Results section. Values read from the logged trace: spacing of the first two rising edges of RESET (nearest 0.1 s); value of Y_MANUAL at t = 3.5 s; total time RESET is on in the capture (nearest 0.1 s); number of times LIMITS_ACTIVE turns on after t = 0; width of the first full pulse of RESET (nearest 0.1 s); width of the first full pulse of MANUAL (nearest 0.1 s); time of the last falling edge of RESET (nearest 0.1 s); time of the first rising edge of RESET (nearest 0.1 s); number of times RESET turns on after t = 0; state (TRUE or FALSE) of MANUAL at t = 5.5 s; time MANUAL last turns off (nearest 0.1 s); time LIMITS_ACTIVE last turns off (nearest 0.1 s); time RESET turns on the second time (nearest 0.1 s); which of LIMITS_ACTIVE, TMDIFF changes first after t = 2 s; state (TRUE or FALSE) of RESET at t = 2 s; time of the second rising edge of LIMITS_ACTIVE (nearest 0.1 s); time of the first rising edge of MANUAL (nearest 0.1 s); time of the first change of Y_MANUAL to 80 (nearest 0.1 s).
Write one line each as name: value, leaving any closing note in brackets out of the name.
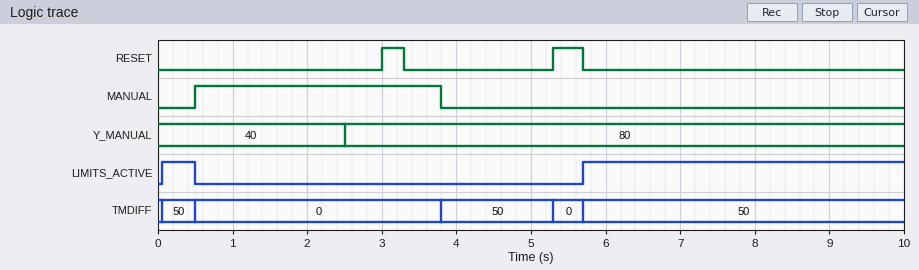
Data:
spacing of the first two rising edges of RESET: 2.3 s
value of Y_MANUAL at t = 3.5 s: 80
total time RESET is on in the capture: 0.7 s
number of times LIMITS_ACTIVE turns on after t = 0: 2
width of the first full pulse of RESET: 0.3 s
width of the first full pulse of MANUAL: 3.3 s
time of the last falling edge of RESET: 5.7 s
time of the first rising edge of RESET: 3.0 s
number of times RESET turns on after t = 0: 2
state (TRUE or FALSE) of MANUAL at t = 5.5 s: FALSE
time MANUAL last turns off: 3.8 s
time LIMITS_ACTIVE last turns off: 0.5 s
time RESET turns on the second time: 5.3 s
which of LIMITS_ACTIVE, TMDIFF changes first after t = 2 s: TMDIFF
state (TRUE or FALSE) of RESET at t = 2 s: FALSE
time of the second rising edge of LIMITS_ACTIVE: 5.7 s
time of the first rising edge of MANUAL: 0.5 s
time of the first change of Y_MANUAL to 80: 2.5 s
